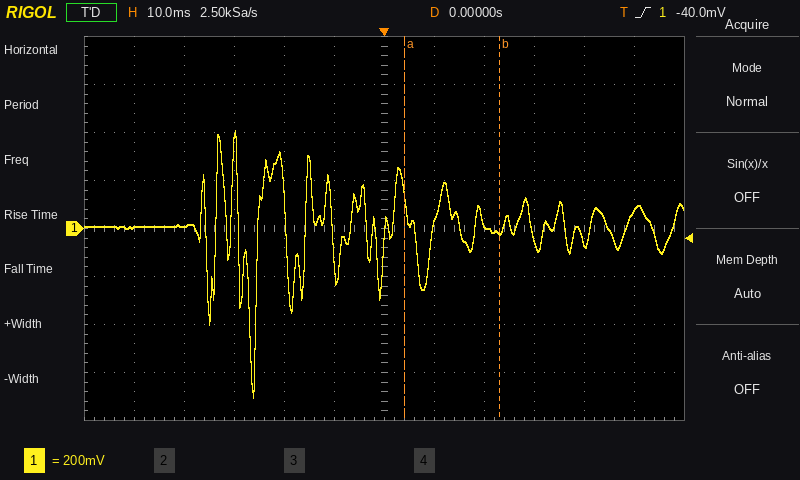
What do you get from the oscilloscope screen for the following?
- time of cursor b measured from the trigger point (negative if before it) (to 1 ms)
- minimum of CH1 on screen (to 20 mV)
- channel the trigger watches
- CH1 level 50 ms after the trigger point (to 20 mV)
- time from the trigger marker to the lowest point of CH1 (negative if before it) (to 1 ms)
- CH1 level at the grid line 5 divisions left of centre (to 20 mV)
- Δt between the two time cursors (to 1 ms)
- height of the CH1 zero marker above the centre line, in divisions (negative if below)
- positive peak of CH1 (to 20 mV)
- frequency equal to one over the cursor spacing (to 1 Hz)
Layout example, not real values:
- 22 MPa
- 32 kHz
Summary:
- +23 ms
- -700 mV
- CH1
- 80 mV
- -26 ms
- 0 mV
- 19 ms
- 0.0 div
- 400 mV
- 53 Hz
